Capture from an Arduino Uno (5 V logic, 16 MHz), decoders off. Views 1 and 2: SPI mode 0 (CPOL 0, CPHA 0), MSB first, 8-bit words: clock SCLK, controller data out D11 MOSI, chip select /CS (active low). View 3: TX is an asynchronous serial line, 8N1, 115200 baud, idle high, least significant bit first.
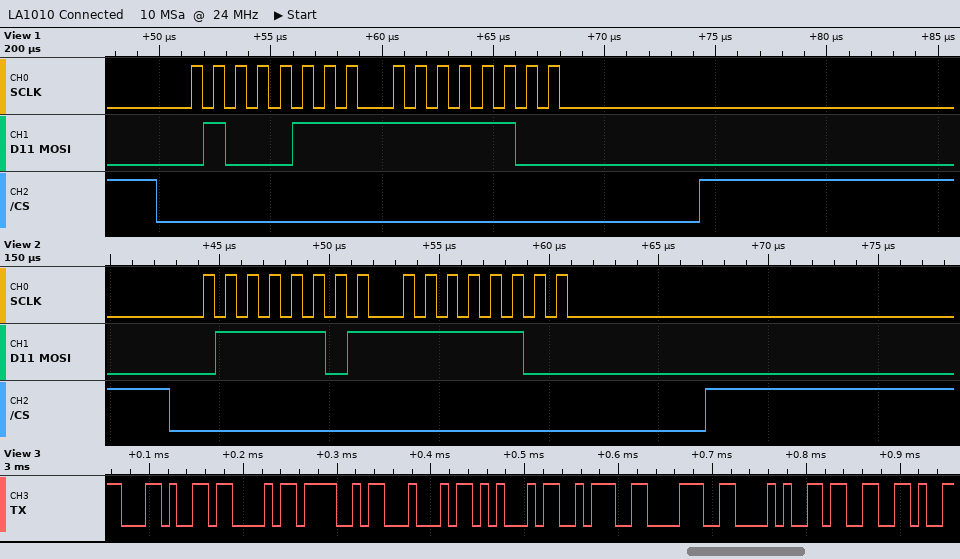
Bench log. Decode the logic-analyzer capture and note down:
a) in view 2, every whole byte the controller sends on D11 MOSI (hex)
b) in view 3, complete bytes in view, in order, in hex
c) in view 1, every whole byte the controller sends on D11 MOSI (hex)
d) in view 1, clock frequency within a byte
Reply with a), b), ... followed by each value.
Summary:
a) 7D FC
b) 2C 43 4F 44 45 3A 38 28 33
c) 47 FC
d) 1 MHz
